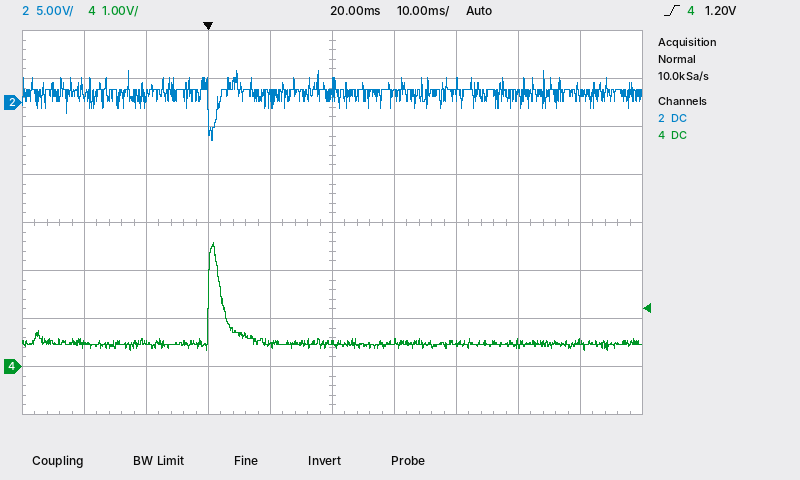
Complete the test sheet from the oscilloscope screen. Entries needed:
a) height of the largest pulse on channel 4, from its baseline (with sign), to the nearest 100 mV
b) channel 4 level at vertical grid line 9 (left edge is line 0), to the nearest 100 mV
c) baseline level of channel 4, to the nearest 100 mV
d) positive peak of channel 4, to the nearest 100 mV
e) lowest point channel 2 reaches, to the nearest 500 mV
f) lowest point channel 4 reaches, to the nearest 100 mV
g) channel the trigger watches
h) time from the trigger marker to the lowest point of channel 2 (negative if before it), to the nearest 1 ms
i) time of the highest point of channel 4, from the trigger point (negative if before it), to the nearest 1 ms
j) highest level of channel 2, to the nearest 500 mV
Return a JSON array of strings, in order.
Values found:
["+2.1 V", "500 mV", "500 mV", "2.6 V", "-4.0 V", "300 mV", "channel 4", "+1 ms", "+1 ms", "3.5 V"]
